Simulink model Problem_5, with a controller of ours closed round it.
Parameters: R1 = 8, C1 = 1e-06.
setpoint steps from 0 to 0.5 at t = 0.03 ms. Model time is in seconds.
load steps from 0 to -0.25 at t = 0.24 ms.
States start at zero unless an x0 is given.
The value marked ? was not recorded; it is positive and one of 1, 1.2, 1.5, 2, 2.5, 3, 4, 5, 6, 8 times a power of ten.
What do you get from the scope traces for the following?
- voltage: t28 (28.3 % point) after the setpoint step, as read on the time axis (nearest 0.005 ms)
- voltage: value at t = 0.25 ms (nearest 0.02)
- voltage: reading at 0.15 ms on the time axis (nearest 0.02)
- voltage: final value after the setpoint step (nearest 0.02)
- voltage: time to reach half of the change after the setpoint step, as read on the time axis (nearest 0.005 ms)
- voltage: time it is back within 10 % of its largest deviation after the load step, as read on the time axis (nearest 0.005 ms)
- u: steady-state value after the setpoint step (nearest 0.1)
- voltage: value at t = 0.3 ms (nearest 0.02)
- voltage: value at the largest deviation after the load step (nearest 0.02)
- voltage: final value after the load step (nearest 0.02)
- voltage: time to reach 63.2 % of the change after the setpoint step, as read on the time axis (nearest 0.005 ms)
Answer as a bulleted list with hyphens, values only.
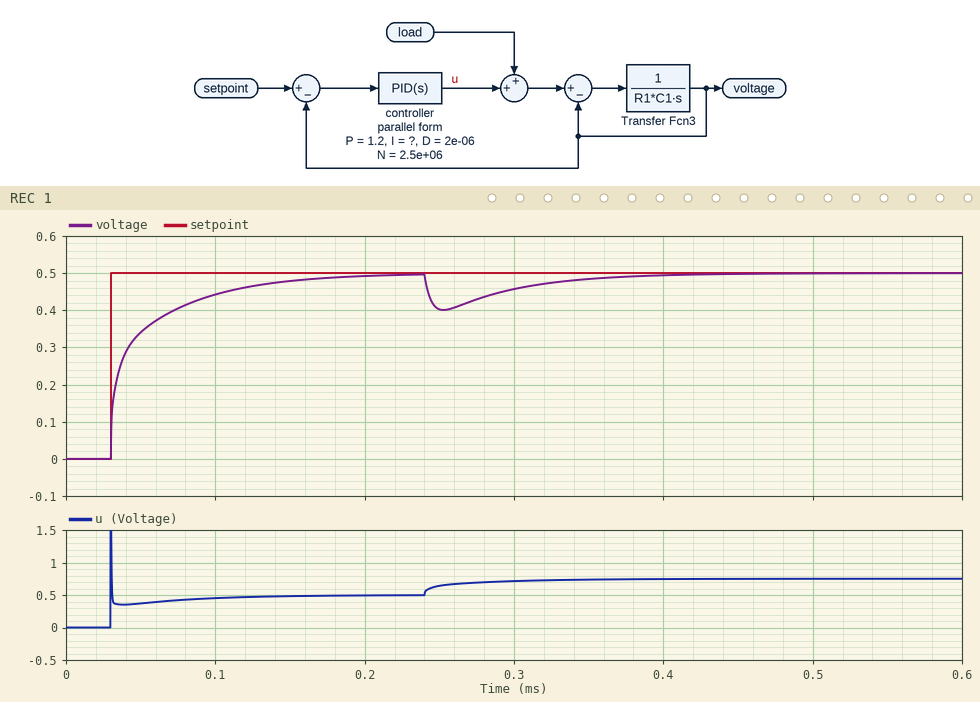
- 0.030 ms
- 0.40
- 0.48
- 0.50
- 0.035 ms
- 0.375 ms
- 0.5
- 0.46
- 0.40
- 0.50
- 0.045 ms
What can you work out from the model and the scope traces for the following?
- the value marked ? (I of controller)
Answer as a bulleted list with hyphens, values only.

- 40000
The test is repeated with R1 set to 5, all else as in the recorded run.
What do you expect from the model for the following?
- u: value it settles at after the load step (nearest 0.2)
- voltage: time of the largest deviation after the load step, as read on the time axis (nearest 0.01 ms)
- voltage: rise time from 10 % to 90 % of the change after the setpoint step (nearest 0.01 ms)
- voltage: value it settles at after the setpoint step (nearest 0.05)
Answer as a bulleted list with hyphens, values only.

- 0.8
- 0.25 ms
- 0.08 ms
- 0.50
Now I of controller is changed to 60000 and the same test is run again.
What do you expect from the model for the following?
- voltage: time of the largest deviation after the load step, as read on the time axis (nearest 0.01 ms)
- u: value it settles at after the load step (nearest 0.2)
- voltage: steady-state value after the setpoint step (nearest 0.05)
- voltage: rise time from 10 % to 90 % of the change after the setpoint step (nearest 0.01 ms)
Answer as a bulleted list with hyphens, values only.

- 0.25 ms
- 0.8
- 0.50
- 0.05 ms
